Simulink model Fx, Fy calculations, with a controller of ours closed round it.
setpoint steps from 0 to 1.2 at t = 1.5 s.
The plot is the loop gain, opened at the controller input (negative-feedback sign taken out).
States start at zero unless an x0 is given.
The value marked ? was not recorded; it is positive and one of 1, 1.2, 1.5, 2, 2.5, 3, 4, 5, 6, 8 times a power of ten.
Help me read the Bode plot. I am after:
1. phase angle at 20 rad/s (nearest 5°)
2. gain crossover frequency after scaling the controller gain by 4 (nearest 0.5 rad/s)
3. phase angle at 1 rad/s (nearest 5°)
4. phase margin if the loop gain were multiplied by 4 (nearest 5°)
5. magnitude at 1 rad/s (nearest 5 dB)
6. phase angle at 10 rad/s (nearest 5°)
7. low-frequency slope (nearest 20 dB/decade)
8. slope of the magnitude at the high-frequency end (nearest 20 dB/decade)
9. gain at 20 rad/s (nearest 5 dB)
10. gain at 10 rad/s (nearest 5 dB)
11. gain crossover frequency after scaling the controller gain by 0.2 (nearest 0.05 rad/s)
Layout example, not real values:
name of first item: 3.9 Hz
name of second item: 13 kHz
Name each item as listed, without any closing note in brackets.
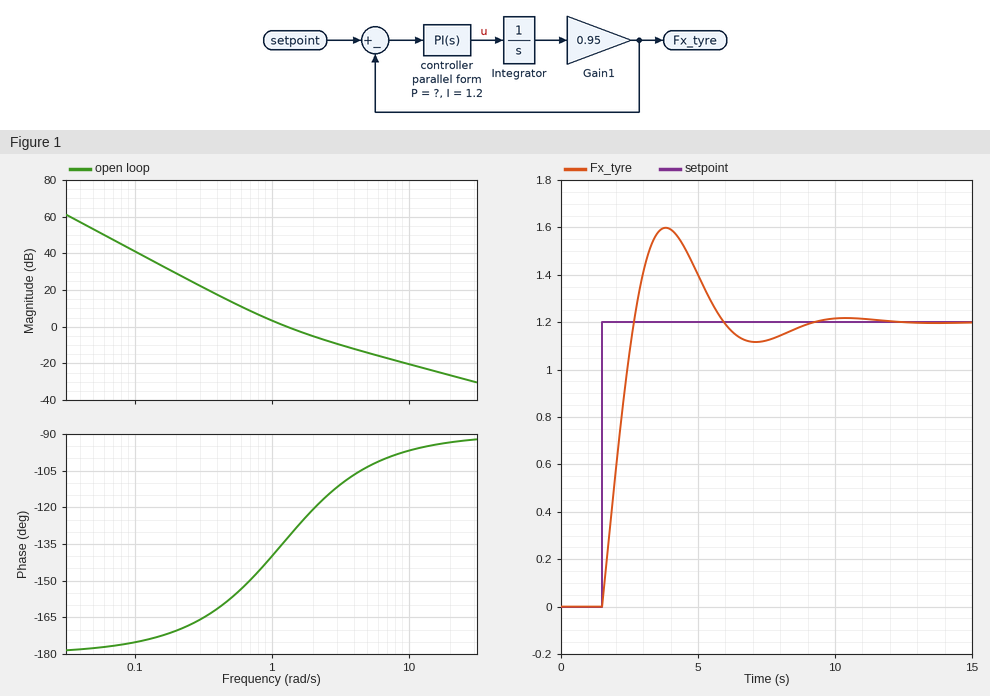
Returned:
phase angle at 20 rad/s: -95°
gain crossover frequency after scaling the controller gain by 4: 4.0 rad/s
phase angle at 1 rad/s: -140°
phase margin if the loop gain were multiplied by 4: 75°
magnitude at 1 rad/s: 5 dB
phase angle at 10 rad/s: -95°
low-frequency slope: -40 dB/decade
slope of the magnitude at the high-frequency end: -20 dB/decade
gain at 20 rad/s: -25 dB
gain at 10 rad/s: -20 dB
gain crossover frequency after scaling the controller gain by 0.2: 0.50 rad/s
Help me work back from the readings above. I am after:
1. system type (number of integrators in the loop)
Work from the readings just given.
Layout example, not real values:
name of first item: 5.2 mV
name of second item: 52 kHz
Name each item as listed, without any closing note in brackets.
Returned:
system type: 2
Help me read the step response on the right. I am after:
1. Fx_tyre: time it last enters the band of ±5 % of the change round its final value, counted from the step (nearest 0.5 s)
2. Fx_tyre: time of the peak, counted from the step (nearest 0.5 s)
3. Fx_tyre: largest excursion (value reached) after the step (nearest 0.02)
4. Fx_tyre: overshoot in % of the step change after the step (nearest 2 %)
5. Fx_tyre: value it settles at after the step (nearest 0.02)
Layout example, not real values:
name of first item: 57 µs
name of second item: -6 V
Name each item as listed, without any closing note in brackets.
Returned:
Fx_tyre: time it last enters the band of ±5 % of the change round its final value, counted from the step: 6.5 s
Fx_tyre: time of the peak, counted from the step: 2.5 s
Fx_tyre: largest excursion (value reached) after the step: 1.60
Fx_tyre: overshoot in % of the step change after the step: 34 %
Fx_tyre: value it settles at after the step: 1.20
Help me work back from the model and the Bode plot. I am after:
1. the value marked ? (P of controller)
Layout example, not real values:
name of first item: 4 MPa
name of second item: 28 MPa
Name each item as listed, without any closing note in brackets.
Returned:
the value marked ?: 1
